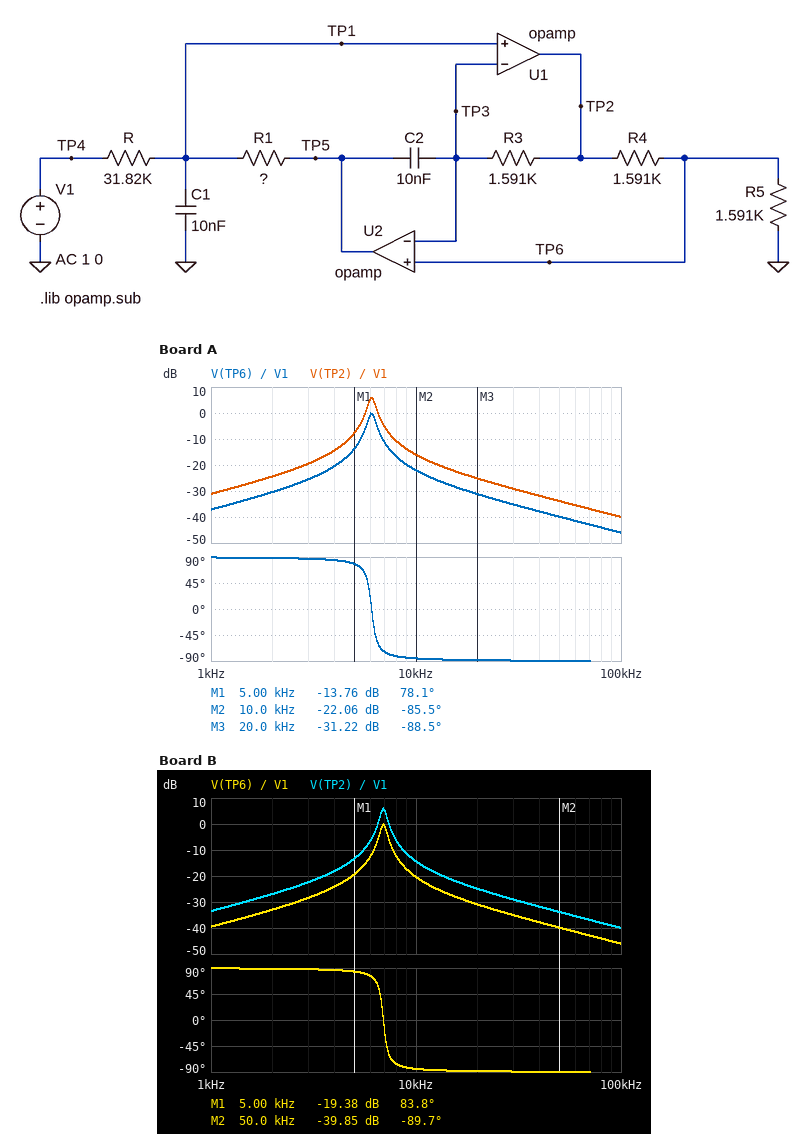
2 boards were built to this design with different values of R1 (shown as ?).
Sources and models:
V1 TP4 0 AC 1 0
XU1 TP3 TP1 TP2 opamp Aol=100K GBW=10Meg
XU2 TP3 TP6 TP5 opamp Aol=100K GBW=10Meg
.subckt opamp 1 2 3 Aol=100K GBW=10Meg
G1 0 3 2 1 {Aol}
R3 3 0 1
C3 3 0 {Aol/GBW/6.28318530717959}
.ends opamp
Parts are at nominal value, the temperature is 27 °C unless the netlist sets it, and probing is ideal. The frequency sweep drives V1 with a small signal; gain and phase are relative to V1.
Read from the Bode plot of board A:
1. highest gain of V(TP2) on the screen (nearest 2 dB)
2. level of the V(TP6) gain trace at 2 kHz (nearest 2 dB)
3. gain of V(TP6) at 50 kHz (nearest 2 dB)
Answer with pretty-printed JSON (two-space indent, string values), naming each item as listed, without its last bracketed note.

{
  "highest gain of V(TP2) on the screen": "6 dB",
  "level of the V(TP6) gain trace at 2 kHz": "-30 dB",
  "gain of V(TP6) at 50 kHz": "-40 dB"
}
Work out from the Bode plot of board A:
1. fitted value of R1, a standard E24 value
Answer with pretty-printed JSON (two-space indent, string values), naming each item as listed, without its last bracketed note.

{
  "fitted value of R1, a standard E24 value": "4.3 kΩ"
}
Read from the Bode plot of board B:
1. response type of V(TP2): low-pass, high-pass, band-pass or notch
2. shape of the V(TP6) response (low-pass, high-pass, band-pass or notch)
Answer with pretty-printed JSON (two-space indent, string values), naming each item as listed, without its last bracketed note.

{
  "response type of V(TP2): low-pass, high-pass, band-pass or notch": "band-pass",
  "shape of the V(TP6) response": "band-pass"
}
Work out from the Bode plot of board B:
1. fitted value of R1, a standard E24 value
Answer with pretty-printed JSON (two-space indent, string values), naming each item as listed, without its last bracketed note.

{
  "fitted value of R1, a standard E24 value": "3.3 kΩ"
}
